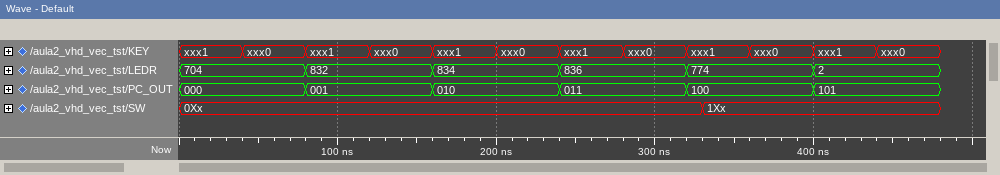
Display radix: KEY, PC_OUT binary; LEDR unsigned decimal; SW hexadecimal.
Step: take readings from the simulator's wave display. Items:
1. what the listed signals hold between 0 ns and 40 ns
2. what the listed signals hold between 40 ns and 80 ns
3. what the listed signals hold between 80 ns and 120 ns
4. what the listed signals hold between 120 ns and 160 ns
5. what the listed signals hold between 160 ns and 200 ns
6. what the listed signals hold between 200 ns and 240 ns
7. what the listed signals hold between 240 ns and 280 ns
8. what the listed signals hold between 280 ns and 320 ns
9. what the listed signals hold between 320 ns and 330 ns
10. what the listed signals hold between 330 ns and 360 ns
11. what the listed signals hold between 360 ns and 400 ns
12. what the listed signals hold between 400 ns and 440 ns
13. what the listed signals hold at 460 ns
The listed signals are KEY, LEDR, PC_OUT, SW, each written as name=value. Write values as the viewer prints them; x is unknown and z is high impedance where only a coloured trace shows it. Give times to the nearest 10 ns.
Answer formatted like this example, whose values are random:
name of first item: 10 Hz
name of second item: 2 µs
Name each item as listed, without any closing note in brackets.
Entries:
what the listed signals hold between 0 ns and 40 ns: KEY=xxx1, LEDR=704, PC_OUT=000, SW=0Xx
what the listed signals hold between 40 ns and 80 ns: KEY=xxx0, LEDR=704, PC_OUT=000, SW=0Xx
what the listed signals hold between 80 ns and 120 ns: KEY=xxx1, LEDR=832, PC_OUT=001, SW=0Xx
what the listed signals hold between 120 ns and 160 ns: KEY=xxx0, LEDR=832, PC_OUT=001, SW=0Xx
what the listed signals hold between 160 ns and 200 ns: KEY=xxx1, LEDR=834, PC_OUT=010, SW=0Xx
what the listed signals hold between 200 ns and 240 ns: KEY=xxx0, LEDR=834, PC_OUT=010, SW=0Xx
what the listed signals hold between 240 ns and 280 ns: KEY=xxx1, LEDR=836, PC_OUT=011, SW=0Xx
what the listed signals hold between 280 ns and 320 ns: KEY=xxx0, LEDR=836, PC_OUT=011, SW=0Xx
what the listed signals hold between 320 ns and 330 ns: KEY=xxx1, LEDR=774, PC_OUT=100, SW=0Xx
what the listed signals hold between 330 ns and 360 ns: KEY=xxx1, LEDR=774, PC_OUT=100, SW=1Xx
what the listed signals hold between 360 ns and 400 ns: KEY=xxx0, LEDR=774, PC_OUT=100, SW=1Xx
what the listed signals hold between 400 ns and 440 ns: KEY=xxx1, LEDR=2, PC_OUT=101, SW=1Xx
what the listed signals hold at 460 ns: KEY=xxx0, LEDR=2, PC_OUT=101, SW=1Xx
